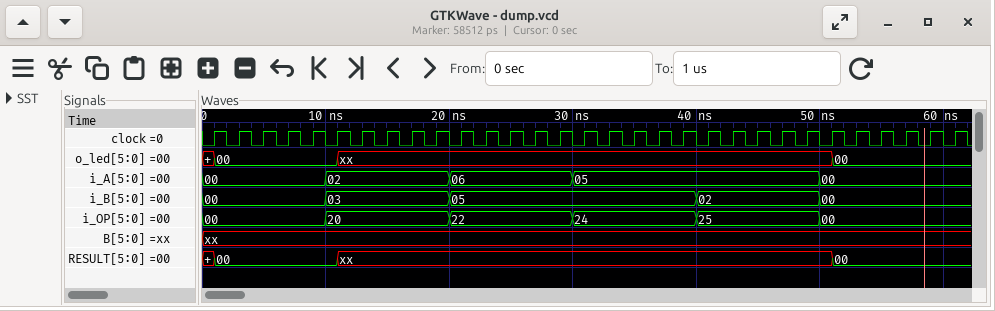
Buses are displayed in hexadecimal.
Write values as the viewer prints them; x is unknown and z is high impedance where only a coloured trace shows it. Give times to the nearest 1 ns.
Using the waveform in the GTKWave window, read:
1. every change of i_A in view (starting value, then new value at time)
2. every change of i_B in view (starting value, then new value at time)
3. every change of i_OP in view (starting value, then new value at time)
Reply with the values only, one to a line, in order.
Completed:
00, 02 at 10 ns, 06 at 20 ns, 05 at 30 ns, 00 at 50 ns
00, 03 at 10 ns, 05 at 20 ns, 02 at 40 ns, 00 at 50 ns
00, 20 at 10 ns, 22 at 20 ns, 24 at 30 ns, 25 at 40 ns, 00 at 50 ns
